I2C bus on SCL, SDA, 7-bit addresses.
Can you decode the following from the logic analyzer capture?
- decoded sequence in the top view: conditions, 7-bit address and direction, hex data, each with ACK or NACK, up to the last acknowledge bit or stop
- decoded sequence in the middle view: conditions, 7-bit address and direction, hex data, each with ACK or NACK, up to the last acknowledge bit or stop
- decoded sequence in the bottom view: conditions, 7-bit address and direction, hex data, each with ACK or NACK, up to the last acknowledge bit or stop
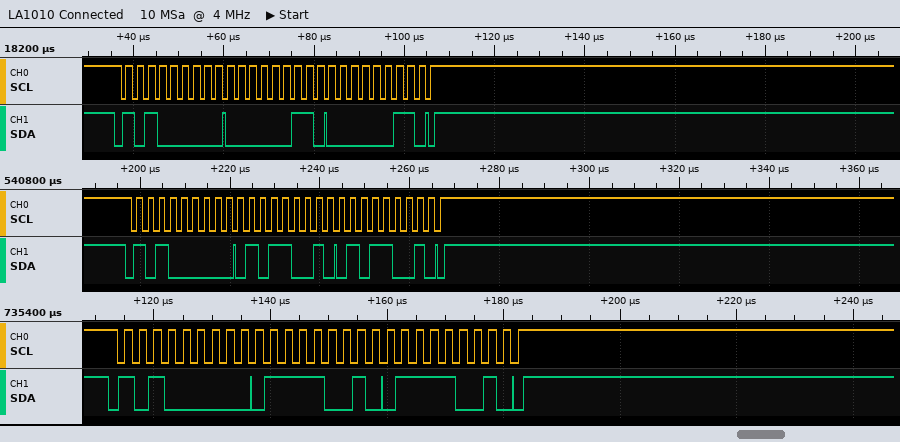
start, address 50 write ACK, 03 ACK, 03 ACK, stop
start, address 50 write ACK, 59 ACK, 59 ACK, stop
start, address 50 write ACK, 79 ACK, 79 ACK, stop
